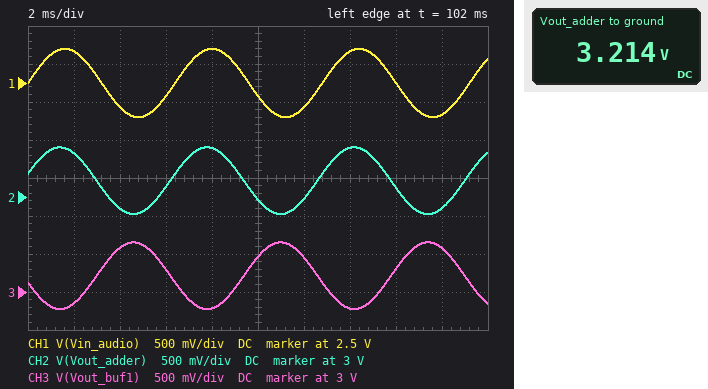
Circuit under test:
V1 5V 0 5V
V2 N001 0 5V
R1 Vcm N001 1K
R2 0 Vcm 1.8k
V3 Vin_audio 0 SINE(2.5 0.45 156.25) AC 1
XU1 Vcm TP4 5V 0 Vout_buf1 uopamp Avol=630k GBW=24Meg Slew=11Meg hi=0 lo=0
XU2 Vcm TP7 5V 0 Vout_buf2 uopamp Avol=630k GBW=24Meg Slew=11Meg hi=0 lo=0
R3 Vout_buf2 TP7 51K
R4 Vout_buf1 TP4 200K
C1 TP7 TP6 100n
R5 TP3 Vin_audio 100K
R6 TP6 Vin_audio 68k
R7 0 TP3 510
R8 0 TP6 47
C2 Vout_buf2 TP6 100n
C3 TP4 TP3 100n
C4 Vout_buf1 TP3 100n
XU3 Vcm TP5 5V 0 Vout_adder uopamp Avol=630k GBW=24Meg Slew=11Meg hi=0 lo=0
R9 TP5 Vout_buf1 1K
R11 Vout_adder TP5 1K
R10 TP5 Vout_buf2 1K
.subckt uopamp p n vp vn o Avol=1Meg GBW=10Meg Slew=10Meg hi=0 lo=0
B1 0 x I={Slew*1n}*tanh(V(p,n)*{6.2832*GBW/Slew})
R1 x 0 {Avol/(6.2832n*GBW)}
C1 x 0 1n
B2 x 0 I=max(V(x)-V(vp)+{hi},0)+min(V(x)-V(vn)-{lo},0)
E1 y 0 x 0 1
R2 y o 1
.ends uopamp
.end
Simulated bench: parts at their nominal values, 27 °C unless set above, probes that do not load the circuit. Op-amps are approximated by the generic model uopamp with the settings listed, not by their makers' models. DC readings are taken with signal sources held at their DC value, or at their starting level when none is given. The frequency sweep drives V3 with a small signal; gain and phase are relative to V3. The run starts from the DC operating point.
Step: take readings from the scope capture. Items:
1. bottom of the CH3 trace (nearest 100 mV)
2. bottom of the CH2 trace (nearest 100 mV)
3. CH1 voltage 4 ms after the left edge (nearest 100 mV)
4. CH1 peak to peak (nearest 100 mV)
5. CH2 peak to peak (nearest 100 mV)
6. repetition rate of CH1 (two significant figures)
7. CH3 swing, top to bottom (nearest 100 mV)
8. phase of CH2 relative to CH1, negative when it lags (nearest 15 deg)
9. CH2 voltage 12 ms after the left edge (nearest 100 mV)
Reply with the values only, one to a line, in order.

2.8 V
2.8 V
2.2 V
900 mV
900 mV
160 Hz
900 mV
15 deg
3.0 V
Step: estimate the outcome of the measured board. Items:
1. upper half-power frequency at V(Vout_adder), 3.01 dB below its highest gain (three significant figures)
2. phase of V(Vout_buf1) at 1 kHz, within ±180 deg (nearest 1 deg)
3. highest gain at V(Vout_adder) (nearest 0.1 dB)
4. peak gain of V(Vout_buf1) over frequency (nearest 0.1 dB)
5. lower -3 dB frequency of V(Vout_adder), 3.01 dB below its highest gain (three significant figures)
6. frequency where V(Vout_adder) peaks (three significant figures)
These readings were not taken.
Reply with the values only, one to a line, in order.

166 Hz
91 deg
0 dB
0 dB
150 Hz
158 Hz
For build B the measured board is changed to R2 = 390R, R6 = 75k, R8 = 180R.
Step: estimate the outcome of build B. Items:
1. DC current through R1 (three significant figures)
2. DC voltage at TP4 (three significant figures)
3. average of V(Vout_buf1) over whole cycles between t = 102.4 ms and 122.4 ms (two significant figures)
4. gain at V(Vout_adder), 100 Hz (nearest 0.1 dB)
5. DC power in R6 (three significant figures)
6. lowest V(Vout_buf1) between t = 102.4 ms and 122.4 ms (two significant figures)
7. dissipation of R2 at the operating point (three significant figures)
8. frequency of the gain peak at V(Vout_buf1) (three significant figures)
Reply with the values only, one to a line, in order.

3.60 mA
1.40 V
1.4 V
-18.9 dB
82.9 µW
960 mV
5.05 mW
158 Hz
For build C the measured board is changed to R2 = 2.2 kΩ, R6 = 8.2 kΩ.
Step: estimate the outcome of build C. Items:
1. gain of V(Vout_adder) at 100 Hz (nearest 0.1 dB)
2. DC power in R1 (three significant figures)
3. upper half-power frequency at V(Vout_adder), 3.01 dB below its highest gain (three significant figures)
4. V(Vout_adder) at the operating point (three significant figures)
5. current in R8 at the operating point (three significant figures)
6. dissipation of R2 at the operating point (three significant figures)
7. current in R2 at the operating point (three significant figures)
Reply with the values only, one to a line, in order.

-18.1 dB
2.44 mW
1.06 kHz
3.44 V
303 µA
5.37 mW
1.56 mA
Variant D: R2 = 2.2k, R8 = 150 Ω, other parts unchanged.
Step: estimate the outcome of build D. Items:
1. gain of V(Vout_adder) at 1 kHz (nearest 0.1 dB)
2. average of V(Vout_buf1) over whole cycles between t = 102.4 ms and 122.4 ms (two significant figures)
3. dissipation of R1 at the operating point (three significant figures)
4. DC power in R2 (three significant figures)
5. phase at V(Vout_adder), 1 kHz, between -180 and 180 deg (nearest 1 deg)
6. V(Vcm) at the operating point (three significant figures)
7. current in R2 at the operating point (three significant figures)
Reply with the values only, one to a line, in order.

-25.8 dB
3.4 V
2.44 mW
5.37 mW
-86 deg
3.44 V
1.56 mA
